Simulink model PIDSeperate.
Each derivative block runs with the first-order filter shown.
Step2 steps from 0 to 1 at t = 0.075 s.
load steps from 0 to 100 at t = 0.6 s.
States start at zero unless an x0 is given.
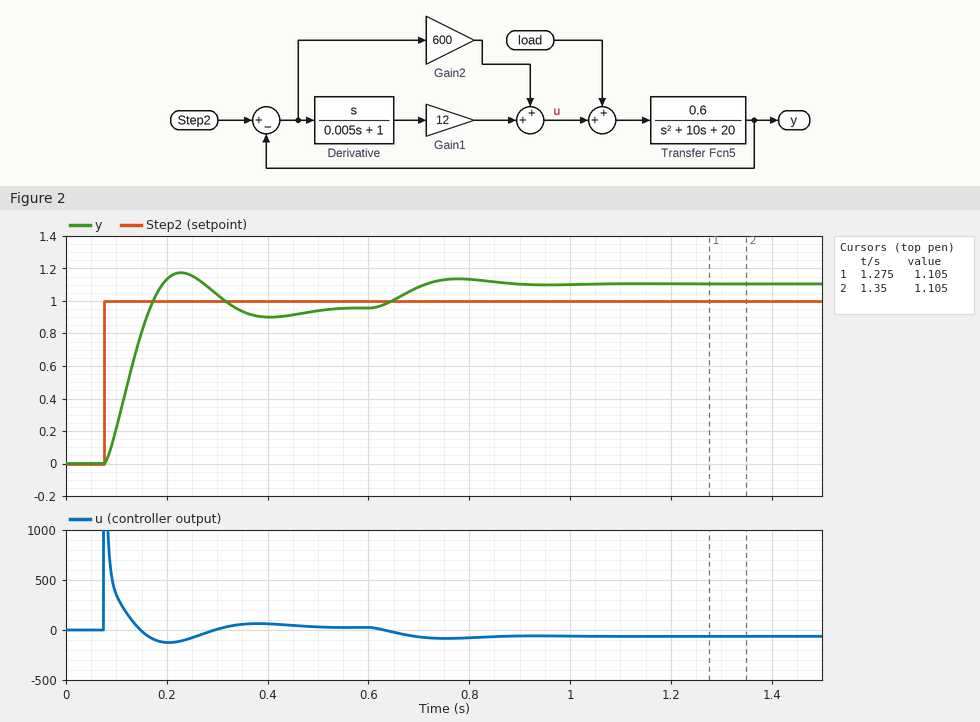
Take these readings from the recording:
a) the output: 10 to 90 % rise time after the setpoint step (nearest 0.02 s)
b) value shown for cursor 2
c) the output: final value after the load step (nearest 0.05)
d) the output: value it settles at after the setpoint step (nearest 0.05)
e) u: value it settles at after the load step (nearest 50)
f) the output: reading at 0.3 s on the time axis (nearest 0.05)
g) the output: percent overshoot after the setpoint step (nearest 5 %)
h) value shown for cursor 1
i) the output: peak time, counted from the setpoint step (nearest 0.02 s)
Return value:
0.06 s
1.105
1.10
0.95
-50
1.05
25 %
1.105
0.16 s
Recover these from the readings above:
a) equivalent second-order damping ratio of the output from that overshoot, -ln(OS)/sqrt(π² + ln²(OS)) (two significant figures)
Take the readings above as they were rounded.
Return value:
0.40
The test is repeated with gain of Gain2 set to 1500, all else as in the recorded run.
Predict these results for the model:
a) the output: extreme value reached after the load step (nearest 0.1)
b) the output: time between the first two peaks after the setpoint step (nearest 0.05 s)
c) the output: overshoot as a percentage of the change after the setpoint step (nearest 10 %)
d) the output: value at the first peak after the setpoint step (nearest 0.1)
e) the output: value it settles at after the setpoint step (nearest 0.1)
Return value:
1.1
0.20 s
40 %
1.4
1.0
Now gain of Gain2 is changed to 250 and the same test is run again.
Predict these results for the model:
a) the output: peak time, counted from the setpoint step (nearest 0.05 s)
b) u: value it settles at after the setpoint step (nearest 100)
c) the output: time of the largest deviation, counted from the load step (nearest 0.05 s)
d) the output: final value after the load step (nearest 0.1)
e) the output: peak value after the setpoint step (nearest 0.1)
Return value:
0.25 s
0
0.30 s
1.2
1.0
